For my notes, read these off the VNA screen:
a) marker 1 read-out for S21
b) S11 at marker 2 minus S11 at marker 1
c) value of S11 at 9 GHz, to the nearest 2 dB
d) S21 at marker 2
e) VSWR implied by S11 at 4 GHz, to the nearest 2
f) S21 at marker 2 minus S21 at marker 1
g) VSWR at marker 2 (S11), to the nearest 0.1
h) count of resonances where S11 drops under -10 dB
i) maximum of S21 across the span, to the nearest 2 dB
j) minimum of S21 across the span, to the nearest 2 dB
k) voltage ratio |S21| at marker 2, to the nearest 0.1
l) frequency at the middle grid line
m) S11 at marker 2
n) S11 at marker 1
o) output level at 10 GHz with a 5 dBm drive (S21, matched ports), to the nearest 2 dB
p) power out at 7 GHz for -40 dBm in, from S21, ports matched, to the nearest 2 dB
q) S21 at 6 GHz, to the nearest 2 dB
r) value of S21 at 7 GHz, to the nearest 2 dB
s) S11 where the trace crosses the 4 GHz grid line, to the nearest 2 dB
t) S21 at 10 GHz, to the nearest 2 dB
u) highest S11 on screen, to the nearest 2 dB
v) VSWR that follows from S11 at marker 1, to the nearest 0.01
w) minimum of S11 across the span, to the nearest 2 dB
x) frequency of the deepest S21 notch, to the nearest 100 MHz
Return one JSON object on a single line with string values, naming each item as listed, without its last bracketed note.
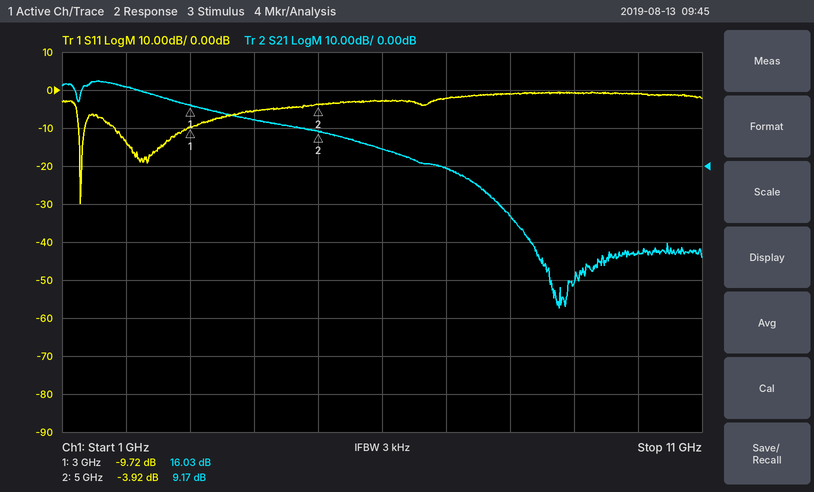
{"marker 1 read-out for S21": "16.03 dB", "S11 at marker 2 minus S11 at marker 1": "5.80 dB", "value of S11 at 9 GHz, to the nearest 2 dB": "0 dB", "S21 at marker 2": "9.17 dB", "VSWR implied by S11 at 4 GHz, to the nearest 2": "4", "S21 at marker 2 minus S21 at marker 1": "-6.86 dB", "VSWR at marker 2 (S11), to the nearest 0.1": "4.5", "count of resonances where S11 drops under -10 dB": "2", "maximum of S21 across the span, to the nearest 2 dB": "22 dB", "minimum of S21 across the span, to the nearest 2 dB": "-38 dB", "voltage ratio |S21| at marker 2, to the nearest 0.1": "2.9", "frequency at the middle grid line": "6 GHz", "S11 at marker 2": "-3.92 dB", "S11 at marker 1": "-9.72 dB", "output level at 10 GHz with a 5 dBm drive (S21, matched ports), to the nearest 2 dB": "-18 dBm", "power out at 7 GHz for -40 dBm in, from S21, ports matched, to the nearest 2 dB": "-40 dBm", "S21 at 6 GHz, to the nearest 2 dB": "4 dB", "value of S21 at 7 GHz, to the nearest 2 dB": "0 dB", "S11 where the trace crosses the 4 GHz grid line, to the nearest 2 dB": "-6 dB", "S21 at 10 GHz, to the nearest 2 dB": "-22 dB", "highest S11 on screen, to the nearest 2 dB": "0 dB", "VSWR that follows from S11 at marker 1, to the nearest 0.01": "1.97", "minimum of S11 across the span, to the nearest 2 dB": "-30 dB", "frequency of the deepest S21 notch, to the nearest 100 MHz": "8.8 GHz"}
